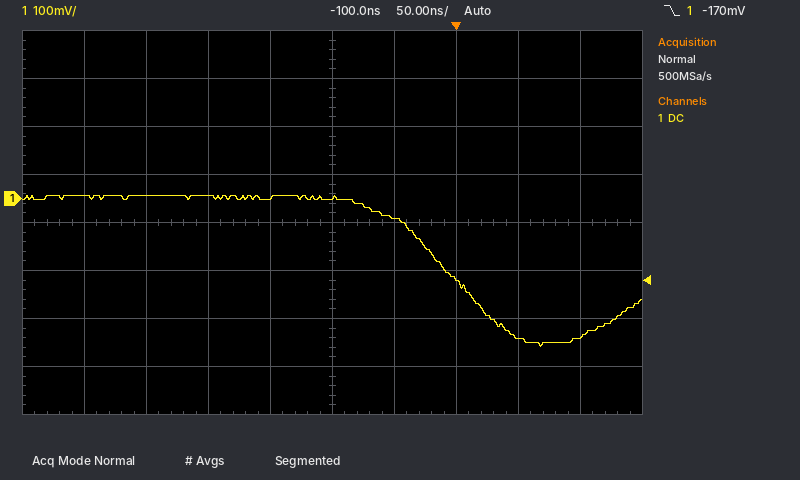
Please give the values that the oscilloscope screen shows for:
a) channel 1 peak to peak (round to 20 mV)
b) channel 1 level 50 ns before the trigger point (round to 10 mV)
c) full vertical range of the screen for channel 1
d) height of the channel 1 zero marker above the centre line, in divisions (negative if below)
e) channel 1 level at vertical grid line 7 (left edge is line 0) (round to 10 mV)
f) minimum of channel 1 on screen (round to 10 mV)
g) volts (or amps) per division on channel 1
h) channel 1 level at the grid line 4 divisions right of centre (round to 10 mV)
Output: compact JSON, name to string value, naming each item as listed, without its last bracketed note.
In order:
{"channel 1 peak to peak": "320 mV", "channel 1 level 50 ns before the trigger point": "-40 mV", "full vertical range of the screen for channel 1": "800 mV", "height of the channel 1 zero marker above the centre line, in divisions": "+0.5 div", "channel 1 level at vertical grid line 7 (left edge is line 0)": "-170 mV", "minimum of channel 1 on screen": "-310 mV", "volts (or amps) per division on channel 1": "100 mV", "channel 1 level at the grid line 4 divisions right of centre": "-290 mV"}
